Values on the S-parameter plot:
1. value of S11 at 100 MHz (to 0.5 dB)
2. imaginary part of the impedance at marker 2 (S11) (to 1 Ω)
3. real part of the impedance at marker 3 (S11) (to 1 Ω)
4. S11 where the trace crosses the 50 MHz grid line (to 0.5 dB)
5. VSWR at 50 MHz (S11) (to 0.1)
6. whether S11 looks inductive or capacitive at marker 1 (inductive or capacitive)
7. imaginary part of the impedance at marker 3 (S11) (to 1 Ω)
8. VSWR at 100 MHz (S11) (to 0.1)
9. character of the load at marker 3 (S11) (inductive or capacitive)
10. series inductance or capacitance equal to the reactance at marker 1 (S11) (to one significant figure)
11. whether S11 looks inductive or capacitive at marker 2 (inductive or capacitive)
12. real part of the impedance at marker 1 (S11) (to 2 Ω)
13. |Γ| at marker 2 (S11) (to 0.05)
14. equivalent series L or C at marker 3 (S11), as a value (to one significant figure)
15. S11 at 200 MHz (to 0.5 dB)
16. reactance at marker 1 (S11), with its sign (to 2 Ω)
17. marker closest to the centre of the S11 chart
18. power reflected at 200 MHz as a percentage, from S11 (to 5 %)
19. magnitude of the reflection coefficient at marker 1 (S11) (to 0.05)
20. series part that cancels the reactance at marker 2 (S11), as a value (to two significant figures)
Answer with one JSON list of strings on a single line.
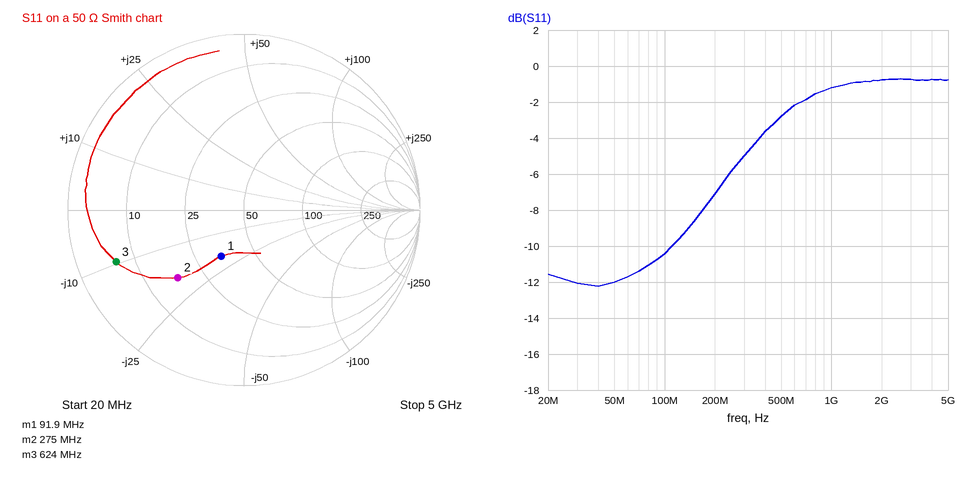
["-10.5 dB", "-19 Ω", "6 Ω", "-12.0 dB", "1.7", "capacitive", "-10 Ω", "1.9", "capacitive", "90 pF", "capacitive", "34 Ω", "0.55", "30 pF", "-7.0 dB", "-20 Ω", "marker 1", "20 %", "0.30", "11 nH"]
